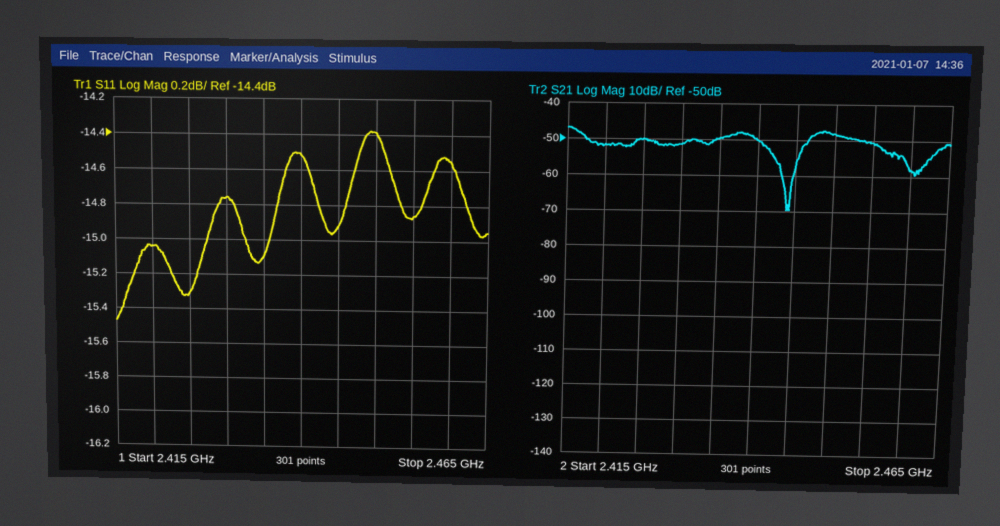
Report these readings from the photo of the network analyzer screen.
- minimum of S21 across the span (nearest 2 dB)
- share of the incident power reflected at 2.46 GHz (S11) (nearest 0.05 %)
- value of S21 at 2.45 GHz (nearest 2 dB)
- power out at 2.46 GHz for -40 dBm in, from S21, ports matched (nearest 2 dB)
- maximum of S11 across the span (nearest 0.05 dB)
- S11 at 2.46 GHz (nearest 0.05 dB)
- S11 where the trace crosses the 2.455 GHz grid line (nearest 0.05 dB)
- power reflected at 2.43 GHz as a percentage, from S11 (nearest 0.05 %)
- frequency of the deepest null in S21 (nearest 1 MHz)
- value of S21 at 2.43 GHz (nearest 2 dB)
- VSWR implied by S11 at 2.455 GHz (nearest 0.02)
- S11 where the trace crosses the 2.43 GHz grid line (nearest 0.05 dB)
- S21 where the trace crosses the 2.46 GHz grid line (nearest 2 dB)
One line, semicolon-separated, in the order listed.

-70 dB; 3.50 %; -48 dB; -98 dBm; -14.40 dB; -14.55 dB; -14.85 dB; 3.35 %; 2.444 GHz; -52 dB; 1.44; -14.75 dB; -58 dB
